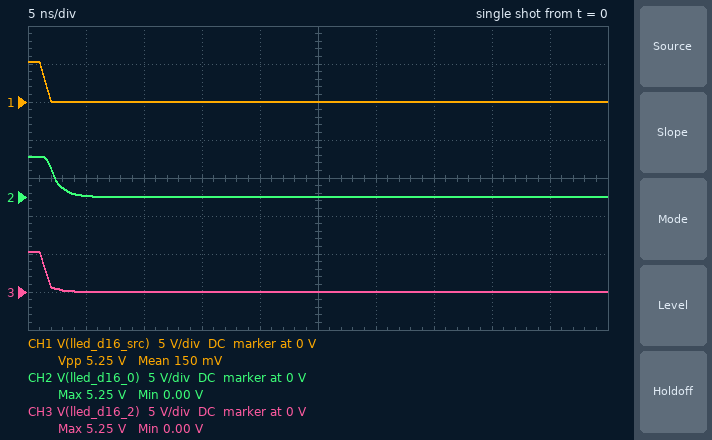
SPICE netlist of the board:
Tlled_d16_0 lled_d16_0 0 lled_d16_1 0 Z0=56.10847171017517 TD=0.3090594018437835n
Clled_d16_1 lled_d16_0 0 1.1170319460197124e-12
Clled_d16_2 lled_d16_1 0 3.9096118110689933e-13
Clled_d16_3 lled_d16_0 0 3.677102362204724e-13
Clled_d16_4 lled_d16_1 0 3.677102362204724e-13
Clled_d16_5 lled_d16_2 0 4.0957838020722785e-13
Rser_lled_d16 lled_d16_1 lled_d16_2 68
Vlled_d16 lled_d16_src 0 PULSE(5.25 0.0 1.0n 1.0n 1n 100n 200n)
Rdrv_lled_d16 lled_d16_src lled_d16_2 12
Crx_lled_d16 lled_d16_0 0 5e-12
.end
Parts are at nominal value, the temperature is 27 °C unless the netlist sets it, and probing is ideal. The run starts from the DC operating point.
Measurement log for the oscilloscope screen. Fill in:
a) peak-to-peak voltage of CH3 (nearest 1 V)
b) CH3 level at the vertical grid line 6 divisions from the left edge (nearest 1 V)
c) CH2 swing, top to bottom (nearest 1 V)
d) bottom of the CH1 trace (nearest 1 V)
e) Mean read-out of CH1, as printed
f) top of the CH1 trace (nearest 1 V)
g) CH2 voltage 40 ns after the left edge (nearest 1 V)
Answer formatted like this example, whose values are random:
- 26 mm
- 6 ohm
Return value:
- 5 V
- 0 V
- 5 V
- 0 V
- 150 mV
- 5 V
- 0 V
